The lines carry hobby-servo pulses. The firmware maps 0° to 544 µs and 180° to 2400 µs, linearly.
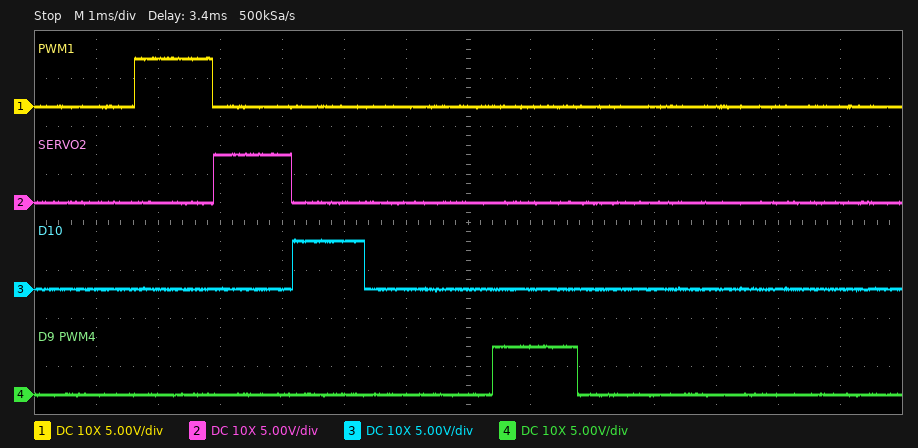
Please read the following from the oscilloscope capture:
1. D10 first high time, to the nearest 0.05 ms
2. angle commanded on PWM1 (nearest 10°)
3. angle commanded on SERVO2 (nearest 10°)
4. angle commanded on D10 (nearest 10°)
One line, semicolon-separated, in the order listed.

1.15 ms; 70°; 70°; 60°
